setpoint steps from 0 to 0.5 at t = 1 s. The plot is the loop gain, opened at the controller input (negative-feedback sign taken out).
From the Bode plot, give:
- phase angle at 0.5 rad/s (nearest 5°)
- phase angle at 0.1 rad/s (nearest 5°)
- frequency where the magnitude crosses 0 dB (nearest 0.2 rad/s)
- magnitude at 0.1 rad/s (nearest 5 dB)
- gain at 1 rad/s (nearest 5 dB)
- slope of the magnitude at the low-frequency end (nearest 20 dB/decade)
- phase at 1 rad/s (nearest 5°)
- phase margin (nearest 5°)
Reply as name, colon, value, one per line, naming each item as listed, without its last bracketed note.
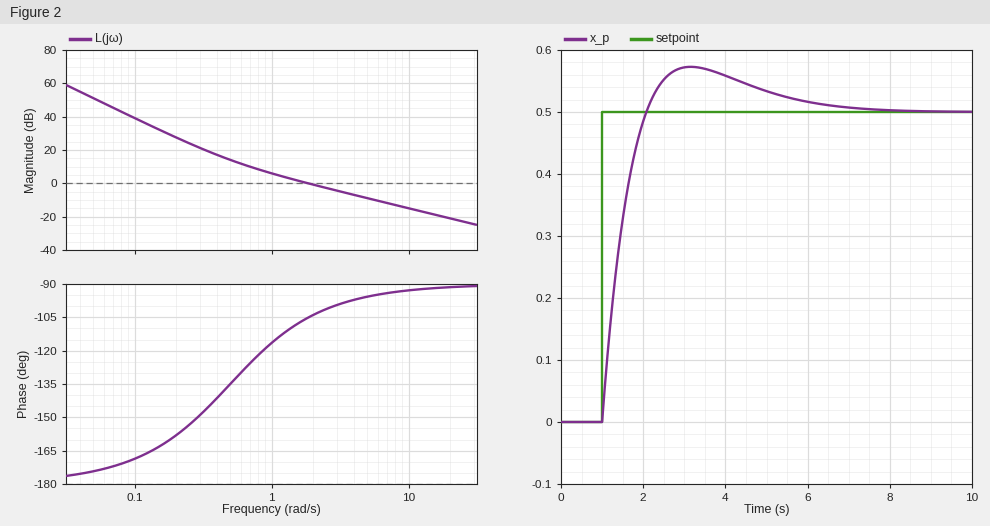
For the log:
phase angle at 0.5 rad/s: -135°
phase angle at 0.1 rad/s: -170°
frequency where the magnitude crosses 0 dB: 1.8 rad/s
magnitude at 0.1 rad/s: 40 dB
gain at 1 rad/s: 5 dB
slope of the magnitude at the low-frequency end: -40 dB/decade
phase at 1 rad/s: -115°
phase margin: 75°
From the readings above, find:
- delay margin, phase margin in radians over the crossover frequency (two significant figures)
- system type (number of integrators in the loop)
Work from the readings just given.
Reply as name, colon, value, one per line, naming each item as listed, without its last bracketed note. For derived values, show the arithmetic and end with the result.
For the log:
delay margin, phase margin in radians over the crossover frequency: 75 × π / 180 / 1.8 = 0.73 s
system type: 2
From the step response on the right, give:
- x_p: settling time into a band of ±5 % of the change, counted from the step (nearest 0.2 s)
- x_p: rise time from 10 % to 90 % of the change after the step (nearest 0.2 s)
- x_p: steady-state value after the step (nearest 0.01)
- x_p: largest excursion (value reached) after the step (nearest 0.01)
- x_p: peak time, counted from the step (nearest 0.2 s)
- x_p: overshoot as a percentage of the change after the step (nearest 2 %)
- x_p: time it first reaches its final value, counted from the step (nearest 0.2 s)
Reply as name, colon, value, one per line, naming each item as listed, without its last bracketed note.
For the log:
x_p: settling time into a band of ±5 % of the change, counted from the step: 4.4 s
x_p: rise time from 10 % to 90 % of the change after the step: 0.8 s
x_p: steady-state value after the step: 0.50
x_p: largest excursion (value reached) after the step: 0.57
x_p: peak time, counted from the step: 2.2 s
x_p: overshoot as a percentage of the change after the step: 14 %
x_p: time it first reaches its final value, counted from the step: 1.0 s
